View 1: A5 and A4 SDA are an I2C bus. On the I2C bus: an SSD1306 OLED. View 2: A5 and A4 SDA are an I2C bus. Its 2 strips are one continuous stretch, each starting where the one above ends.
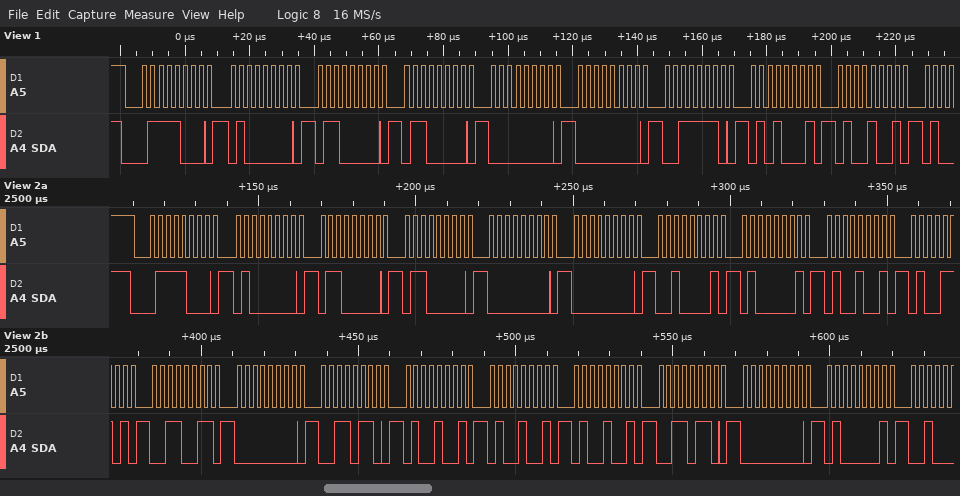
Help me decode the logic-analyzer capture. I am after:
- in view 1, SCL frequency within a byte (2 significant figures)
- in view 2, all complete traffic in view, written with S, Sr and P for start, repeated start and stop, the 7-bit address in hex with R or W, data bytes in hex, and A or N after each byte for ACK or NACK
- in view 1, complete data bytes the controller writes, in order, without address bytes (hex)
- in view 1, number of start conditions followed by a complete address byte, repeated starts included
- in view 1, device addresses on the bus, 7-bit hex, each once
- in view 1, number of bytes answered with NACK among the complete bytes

400 kHz
S 3CW A 40 A 60 A 60 A 00 A 00 A 21 A 41 A 49 A 4D A 33 A 00 A 36 A 49 A 49 A 49 A 36 A 00 A 41 A
40 60 60 00 00 3E 51 49
1
0x3C
0
